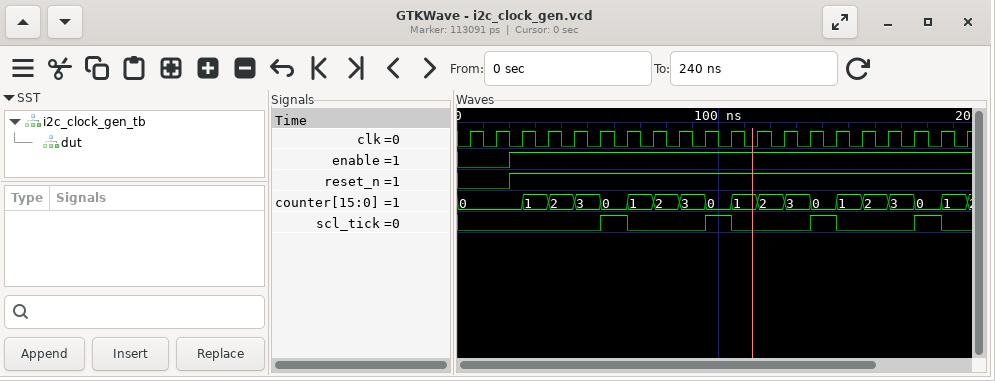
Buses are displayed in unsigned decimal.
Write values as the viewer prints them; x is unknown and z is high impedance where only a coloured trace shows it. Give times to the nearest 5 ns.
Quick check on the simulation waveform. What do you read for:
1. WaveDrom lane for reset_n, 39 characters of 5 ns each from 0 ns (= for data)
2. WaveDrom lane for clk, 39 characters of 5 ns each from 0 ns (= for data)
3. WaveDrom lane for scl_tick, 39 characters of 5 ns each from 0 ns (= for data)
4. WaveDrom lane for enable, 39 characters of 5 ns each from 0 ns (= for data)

{name: 'reset_n', wave: '0...1..................................'}
{name: 'clk', wave: '010101010101010101010101010101010101010'}
{name: 'scl_tick', wave: '0..........1.0.....1.0.....1.0.....1.0.'}
{name: 'enable', wave: '0...1..................................'}
